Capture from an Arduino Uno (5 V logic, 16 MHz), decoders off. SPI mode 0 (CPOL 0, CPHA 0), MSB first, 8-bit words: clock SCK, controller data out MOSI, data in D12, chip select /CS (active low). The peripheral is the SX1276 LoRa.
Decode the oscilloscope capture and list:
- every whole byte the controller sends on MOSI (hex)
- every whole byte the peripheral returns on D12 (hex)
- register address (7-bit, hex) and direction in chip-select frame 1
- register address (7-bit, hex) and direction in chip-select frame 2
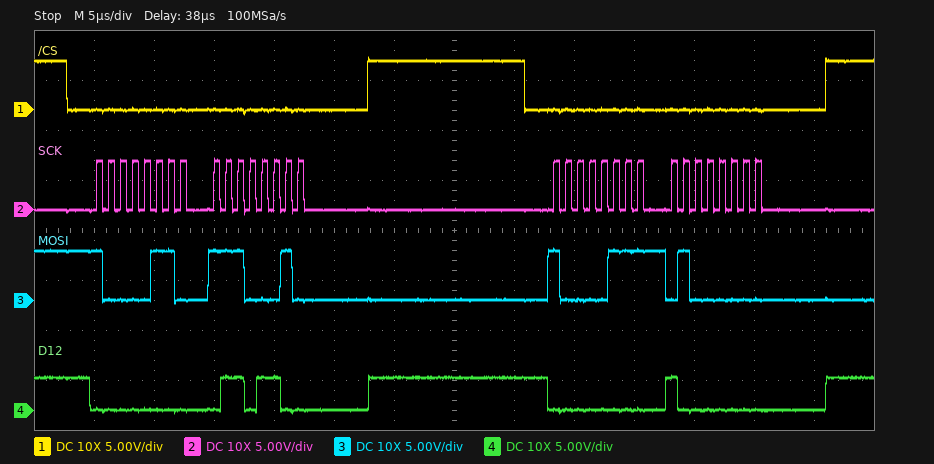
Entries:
86 E2 87 40
00 6C 00 80
0x06 write
0x07 write
